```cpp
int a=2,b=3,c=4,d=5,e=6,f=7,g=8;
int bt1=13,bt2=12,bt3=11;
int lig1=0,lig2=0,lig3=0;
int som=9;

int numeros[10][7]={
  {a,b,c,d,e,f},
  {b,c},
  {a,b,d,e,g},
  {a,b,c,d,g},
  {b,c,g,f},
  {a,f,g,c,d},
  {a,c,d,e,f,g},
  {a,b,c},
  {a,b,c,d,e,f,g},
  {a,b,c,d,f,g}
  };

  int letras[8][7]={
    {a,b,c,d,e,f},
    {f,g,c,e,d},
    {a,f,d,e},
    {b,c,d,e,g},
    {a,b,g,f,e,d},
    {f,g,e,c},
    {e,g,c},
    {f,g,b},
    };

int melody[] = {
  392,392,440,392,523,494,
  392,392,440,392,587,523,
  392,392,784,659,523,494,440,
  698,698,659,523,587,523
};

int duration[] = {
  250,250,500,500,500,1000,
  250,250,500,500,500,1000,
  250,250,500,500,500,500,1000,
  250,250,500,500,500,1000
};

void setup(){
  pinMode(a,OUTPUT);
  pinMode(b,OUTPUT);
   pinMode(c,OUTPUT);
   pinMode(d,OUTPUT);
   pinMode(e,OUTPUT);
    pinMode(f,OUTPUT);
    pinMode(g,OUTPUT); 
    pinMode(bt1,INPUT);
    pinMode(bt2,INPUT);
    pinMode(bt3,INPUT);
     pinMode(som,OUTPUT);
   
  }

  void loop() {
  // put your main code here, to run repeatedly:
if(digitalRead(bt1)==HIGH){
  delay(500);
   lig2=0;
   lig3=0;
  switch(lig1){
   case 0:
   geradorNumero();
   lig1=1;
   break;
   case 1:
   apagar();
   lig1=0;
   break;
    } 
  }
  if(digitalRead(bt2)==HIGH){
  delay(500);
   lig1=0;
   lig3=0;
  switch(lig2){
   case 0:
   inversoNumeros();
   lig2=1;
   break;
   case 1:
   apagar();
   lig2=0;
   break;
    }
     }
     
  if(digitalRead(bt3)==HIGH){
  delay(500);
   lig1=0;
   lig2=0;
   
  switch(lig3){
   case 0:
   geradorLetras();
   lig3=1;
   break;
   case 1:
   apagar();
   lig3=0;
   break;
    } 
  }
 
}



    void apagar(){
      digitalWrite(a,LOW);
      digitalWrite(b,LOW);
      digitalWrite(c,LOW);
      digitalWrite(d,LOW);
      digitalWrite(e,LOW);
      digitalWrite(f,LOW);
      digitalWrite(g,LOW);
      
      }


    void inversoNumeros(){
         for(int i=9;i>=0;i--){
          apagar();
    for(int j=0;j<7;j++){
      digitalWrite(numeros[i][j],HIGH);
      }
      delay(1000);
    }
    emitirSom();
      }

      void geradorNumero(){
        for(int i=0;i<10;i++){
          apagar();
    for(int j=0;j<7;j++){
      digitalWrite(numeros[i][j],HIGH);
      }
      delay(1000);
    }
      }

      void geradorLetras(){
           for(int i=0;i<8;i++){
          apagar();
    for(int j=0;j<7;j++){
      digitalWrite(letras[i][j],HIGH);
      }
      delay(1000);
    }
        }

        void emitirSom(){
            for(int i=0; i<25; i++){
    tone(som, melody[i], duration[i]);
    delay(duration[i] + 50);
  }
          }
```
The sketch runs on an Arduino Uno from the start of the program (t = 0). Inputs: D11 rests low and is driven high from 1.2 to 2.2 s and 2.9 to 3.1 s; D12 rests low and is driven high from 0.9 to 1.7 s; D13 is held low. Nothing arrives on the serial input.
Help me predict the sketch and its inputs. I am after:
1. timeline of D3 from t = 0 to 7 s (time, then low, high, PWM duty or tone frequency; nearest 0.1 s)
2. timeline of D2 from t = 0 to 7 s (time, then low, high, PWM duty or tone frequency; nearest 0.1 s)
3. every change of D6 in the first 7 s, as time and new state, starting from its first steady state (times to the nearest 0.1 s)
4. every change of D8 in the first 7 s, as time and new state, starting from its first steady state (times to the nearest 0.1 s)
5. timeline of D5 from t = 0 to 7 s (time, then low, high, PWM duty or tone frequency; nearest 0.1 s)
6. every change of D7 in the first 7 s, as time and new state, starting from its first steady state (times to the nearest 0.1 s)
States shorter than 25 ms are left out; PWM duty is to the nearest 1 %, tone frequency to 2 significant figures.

0 s low; 1.4 s high; 4.4 s low; 6.4 s high
0 s low; 1.4 s high; 6.4 s low
0 s low; 2.4 s high; 3.4 s low; 4.4 s high; 5.4 s low
0 s low; 1.4 s high; 3.4 s low; 4.4 s high
0 s low; 1.4 s high; 3.4 s low; 4.4 s high; 6.4 s low
0 s low; 1.4 s high; 3.4 s low; 4.4 s high
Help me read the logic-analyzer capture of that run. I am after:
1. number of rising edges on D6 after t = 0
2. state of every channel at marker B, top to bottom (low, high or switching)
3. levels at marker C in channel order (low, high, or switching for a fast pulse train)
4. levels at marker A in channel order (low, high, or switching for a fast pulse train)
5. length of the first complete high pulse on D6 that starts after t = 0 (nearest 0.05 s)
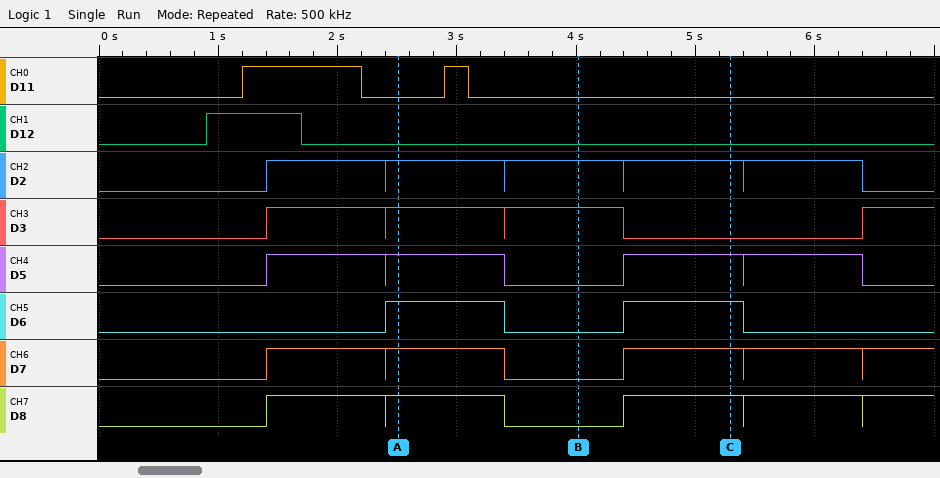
2
D11 low, D12 low, D2 high, D3 high, D5 low, D6 low, D7 low, D8 low
D11 low, D12 low, D2 high, D3 low, D5 high, D6 high, D7 high, D8 high
D11 low, D12 low, D2 high, D3 high, D5 high, D6 high, D7 high, D8 high
1.00 s
